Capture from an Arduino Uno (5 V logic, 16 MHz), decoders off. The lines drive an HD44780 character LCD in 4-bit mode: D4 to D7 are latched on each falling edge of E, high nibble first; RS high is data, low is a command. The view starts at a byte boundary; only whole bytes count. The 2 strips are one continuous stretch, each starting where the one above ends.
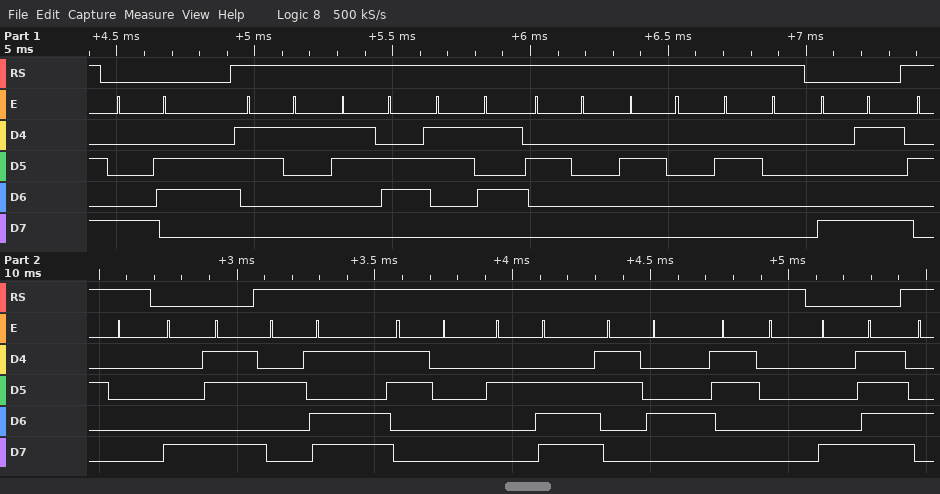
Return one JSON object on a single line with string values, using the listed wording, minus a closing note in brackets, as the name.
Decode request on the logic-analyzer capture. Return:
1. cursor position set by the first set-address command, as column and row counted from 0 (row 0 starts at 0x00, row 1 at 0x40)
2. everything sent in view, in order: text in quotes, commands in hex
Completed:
{"cursor position set by the first set-address command, as column and row counted from 0": "column 6, row 0", "everything sent in view, in order: text in quotes, commands in hex": "0x86 \"165   \" 0x89 \" \" 0x8B \"-0.40\" 0x8F"}
